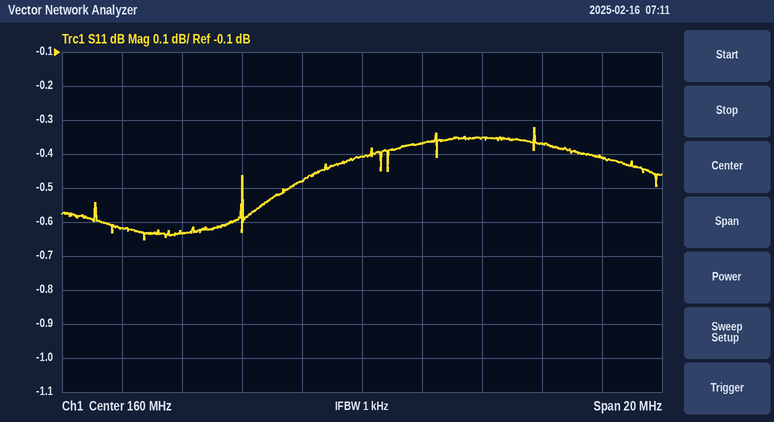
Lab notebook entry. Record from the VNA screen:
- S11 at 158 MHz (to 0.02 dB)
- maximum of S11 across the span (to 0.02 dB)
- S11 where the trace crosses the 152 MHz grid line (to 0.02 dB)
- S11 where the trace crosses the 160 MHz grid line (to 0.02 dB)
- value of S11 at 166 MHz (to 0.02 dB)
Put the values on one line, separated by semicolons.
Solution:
-0.48 dB; -0.32 dB; -0.62 dB; -0.40 dB; -0.36 dB
